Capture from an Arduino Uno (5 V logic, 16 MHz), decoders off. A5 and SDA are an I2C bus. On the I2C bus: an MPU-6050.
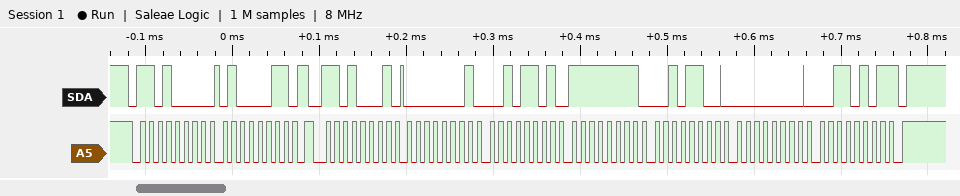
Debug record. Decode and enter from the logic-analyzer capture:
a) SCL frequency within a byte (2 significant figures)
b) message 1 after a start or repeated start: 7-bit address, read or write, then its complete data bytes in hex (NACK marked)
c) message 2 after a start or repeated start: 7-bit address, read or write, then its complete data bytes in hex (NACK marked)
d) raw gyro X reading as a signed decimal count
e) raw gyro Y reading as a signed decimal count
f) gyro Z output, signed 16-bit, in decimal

100 kHz
0x68 write: 43
0x68 read: 01 2D FF 2C 00 35 NACK
301
-212
53
